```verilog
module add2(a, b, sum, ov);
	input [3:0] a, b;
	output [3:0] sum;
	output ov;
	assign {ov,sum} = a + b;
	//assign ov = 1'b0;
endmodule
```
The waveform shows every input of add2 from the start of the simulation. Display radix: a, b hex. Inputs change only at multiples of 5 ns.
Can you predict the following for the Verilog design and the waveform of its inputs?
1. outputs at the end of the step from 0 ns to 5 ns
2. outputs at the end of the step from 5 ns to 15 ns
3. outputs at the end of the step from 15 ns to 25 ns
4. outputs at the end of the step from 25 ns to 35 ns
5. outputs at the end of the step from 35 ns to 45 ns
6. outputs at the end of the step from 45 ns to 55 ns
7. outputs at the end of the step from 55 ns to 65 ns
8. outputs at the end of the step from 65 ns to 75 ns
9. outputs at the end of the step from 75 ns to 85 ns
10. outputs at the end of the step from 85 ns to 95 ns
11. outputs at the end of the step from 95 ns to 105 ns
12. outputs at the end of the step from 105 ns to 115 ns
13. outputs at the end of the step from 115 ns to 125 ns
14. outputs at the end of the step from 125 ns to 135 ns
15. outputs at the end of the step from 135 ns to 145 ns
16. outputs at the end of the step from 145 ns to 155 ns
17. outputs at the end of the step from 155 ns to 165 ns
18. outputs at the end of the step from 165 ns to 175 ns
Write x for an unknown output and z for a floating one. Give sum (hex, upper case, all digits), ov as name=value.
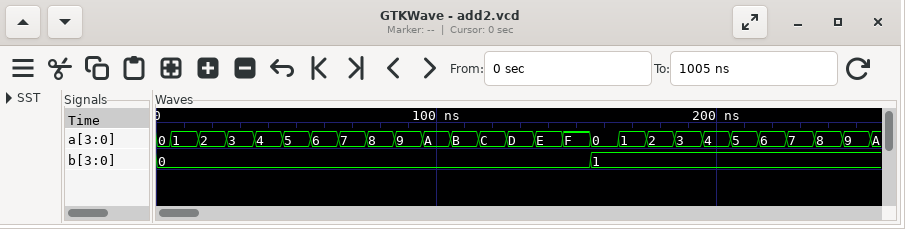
sum=0, ov=0
sum=1, ov=0
sum=2, ov=0
sum=3, ov=0
sum=4, ov=0
sum=5, ov=0
sum=6, ov=0
sum=7, ov=0
sum=8, ov=0
sum=9, ov=0
sum=A, ov=0
sum=B, ov=0
sum=C, ov=0
sum=D, ov=0
sum=E, ov=0
sum=F, ov=0
sum=1, ov=0
sum=2, ov=0
